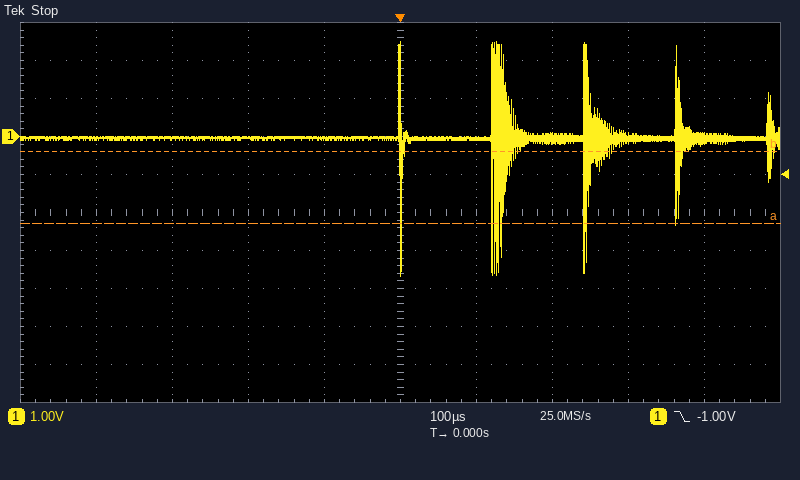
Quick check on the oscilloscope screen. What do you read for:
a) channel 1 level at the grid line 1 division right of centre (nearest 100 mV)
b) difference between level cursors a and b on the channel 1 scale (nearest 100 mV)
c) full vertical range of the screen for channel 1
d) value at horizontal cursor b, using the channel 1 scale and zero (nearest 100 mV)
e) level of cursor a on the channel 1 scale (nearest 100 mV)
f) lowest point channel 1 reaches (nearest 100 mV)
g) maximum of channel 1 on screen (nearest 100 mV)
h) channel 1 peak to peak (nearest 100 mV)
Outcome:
0.0 V
1.9 V
10 V
-400 mV
-2.3 V
-3.7 V
2.5 V
6.2 V
